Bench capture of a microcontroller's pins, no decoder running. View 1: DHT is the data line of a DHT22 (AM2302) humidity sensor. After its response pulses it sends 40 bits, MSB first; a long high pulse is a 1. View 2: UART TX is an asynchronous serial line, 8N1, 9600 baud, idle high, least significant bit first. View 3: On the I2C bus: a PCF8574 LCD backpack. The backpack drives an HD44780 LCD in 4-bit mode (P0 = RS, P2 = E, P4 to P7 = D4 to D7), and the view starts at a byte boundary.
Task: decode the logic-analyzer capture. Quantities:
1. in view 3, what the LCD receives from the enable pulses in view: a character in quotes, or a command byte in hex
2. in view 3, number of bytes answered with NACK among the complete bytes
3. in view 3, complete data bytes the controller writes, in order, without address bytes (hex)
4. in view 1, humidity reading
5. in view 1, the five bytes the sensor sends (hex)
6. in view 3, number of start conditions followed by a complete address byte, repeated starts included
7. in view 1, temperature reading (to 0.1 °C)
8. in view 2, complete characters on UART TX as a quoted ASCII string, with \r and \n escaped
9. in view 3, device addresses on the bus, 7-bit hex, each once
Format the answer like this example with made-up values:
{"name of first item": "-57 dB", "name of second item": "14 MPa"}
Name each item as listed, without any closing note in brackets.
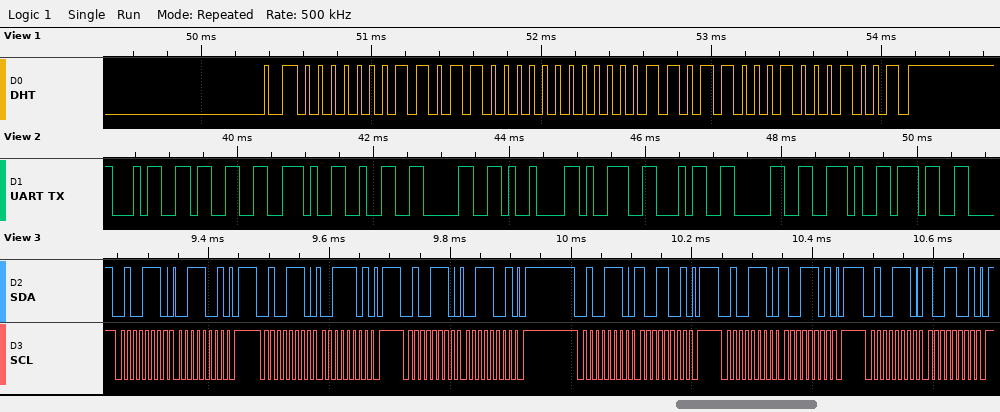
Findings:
{"in view 3, what the LCD receives from the enable pulses in view: a character in quotes, or a command byte in hex": "'9'", "in view 3, number of bytes answered with NACK among the complete bytes": "0", "in view 3, complete data bytes the controller writes, in order, without address bytes": "39 3D 39 99 9D 99", "in view 1, humidity reading": "43.2 %", "in view 1, the five bytes the sensor sends": "01 B0 00 D8 89", "in view 3, number of start conditions followed by a complete address byte, repeated starts included": "6", "in view 1, temperature reading": "21.6 °C", "in view 2, complete characters on UART TX as a quoted ASCII string, with \\r and \\n escaped": "\"43.20\\t940.7\"", "in view 3, device addresses on the bus, 7-bit hex, each once": "0x27"}
